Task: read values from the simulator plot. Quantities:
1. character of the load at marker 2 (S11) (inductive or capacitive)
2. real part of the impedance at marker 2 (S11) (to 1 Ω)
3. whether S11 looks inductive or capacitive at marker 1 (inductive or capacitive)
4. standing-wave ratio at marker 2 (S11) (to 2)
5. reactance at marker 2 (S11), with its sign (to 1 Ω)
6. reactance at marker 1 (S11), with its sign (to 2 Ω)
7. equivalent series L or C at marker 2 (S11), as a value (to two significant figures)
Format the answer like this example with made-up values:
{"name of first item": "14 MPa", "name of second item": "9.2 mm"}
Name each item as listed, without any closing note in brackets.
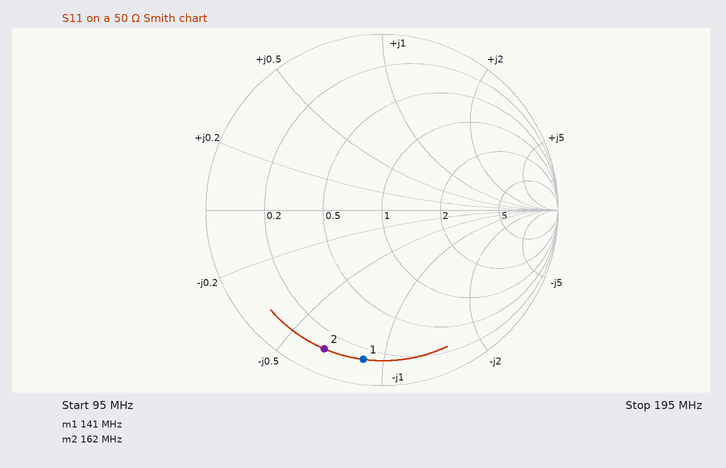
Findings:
{"character of the load at marker 2 (S11)": "capacitive", "real part of the impedance at marker 2 (S11)": "6 Ω", "whether S11 looks inductive or capacitive at marker 1": "capacitive", "standing-wave ratio at marker 2 (S11)": "12", "reactance at marker 2 (S11), with its sign": "-33 Ω", "reactance at marker 1 (S11), with its sign": "-44 Ω", "equivalent series L or C at marker 2 (S11), as a value": "30 pF"}
